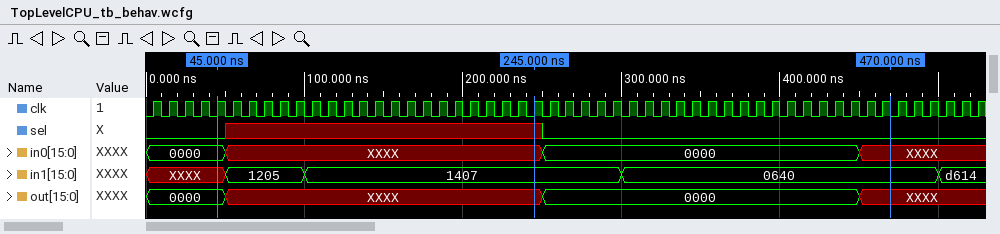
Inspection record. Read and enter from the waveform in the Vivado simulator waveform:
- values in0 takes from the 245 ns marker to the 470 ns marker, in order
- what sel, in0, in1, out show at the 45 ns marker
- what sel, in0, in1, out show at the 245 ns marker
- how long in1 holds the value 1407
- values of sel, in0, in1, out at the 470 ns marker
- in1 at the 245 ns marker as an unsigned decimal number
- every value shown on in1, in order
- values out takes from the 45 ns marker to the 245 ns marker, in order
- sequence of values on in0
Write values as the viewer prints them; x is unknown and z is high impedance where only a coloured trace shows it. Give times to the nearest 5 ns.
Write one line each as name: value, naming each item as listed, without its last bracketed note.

values in0 takes from the 245 ns marker to the 470 ns marker, in order: XXXX, 0000, XXXX
what sel, in0, in1, out show at the 45 ns marker: sel=0, in0=0000, in1=XXXX, out=0000
what sel, in0, in1, out show at the 245 ns marker: sel=x, in0=XXXX, in1=1407, out=XXXX
how long in1 holds the value 1407: 200 ns
values of sel, in0, in1, out at the 470 ns marker: sel=0, in0=XXXX, in1=0640, out=XXXX
in1 at the 245 ns marker as an unsigned decimal number: 5127
every value shown on in1, in order: XXXX, 1205, 1407, 0640, d614
values out takes from the 45 ns marker to the 245 ns marker, in order: 0000, XXXX
sequence of values on in0: 0000, XXXX, 0000, XXXX
